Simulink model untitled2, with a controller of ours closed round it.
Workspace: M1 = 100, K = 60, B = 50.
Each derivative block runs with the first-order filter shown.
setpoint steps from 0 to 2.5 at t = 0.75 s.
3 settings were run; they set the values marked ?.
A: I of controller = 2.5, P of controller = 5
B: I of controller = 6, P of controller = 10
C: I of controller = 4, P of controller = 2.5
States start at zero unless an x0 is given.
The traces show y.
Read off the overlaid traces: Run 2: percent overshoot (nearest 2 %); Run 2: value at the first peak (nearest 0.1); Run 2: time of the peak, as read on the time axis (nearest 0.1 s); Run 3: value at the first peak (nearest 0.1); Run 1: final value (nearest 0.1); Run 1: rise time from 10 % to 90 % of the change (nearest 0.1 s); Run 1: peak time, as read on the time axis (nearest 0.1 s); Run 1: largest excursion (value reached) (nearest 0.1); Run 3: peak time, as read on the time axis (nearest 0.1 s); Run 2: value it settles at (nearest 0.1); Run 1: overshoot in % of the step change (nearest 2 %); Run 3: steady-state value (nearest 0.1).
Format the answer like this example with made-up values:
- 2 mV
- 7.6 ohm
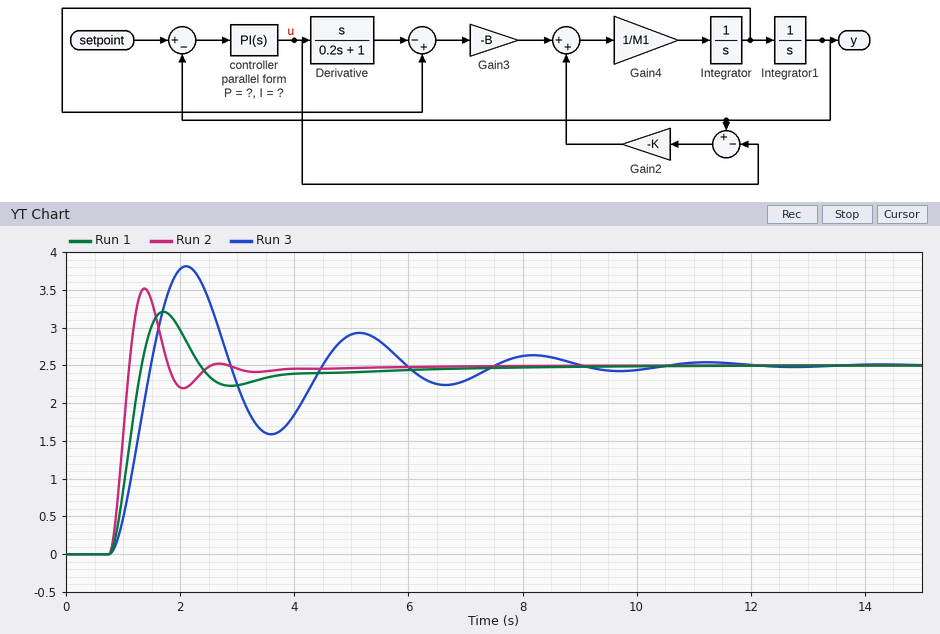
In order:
- 40 %
- 3.5
- 1.4 s
- 3.8
- 2.5
- 0.4 s
- 1.7 s
- 3.2
- 2.1 s
- 2.5
- 28 %
- 2.5
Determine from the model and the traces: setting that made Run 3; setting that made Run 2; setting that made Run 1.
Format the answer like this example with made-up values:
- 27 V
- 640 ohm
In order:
- C
- B
- A
